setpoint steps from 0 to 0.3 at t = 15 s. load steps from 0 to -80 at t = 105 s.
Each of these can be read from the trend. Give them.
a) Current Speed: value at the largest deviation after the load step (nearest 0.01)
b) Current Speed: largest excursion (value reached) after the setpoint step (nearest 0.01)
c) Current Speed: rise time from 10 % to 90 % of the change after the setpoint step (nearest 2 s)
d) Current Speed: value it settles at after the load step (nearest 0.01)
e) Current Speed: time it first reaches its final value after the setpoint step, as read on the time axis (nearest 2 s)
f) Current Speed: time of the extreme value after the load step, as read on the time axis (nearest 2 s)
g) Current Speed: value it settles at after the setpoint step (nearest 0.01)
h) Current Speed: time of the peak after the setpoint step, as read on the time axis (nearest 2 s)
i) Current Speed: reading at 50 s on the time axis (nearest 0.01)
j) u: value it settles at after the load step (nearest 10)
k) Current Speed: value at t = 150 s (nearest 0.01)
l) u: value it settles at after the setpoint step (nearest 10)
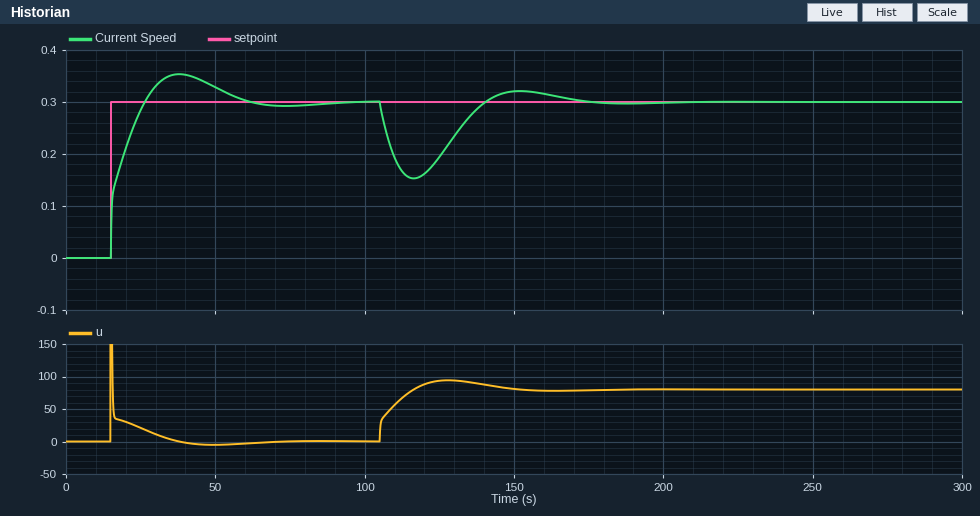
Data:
0.15
0.35
8 s
0.30
26 s
116 s
0.30
38 s
0.33
80
0.32
0
